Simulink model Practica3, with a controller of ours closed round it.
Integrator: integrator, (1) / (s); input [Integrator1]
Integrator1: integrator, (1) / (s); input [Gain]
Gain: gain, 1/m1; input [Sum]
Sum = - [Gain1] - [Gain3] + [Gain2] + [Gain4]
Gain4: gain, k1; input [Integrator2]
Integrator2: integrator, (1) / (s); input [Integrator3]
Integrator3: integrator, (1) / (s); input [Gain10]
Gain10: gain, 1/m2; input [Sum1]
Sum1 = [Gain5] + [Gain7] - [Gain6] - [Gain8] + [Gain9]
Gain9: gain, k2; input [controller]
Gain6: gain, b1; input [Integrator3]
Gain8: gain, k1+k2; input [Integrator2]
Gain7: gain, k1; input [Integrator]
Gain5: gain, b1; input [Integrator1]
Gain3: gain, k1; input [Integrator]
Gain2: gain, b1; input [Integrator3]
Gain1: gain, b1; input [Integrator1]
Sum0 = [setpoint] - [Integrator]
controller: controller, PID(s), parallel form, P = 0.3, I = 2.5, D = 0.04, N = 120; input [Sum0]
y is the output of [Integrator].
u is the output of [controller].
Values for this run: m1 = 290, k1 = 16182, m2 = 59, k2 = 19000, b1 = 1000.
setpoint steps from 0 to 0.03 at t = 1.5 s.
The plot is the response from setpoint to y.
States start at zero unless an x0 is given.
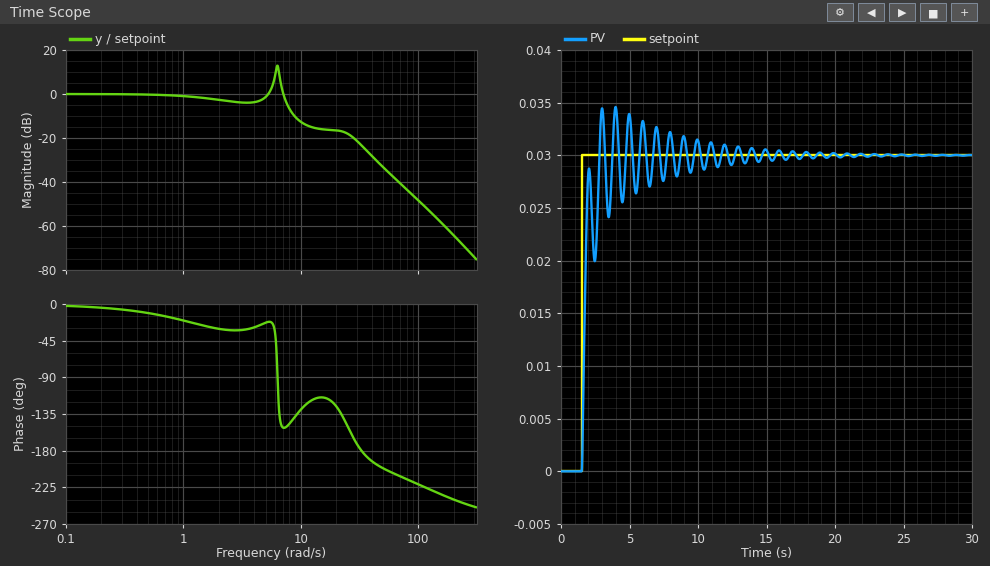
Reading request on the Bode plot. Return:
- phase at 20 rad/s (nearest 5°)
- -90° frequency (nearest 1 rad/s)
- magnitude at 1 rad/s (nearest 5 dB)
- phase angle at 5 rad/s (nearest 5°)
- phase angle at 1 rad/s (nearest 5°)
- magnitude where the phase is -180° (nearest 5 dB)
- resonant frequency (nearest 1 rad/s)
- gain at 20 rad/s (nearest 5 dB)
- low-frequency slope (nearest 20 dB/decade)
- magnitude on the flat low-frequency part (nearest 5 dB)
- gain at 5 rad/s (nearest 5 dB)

-125°
6 rad/s
0 dB
-25°
-20°
-25 dB
6 rad/s
-15 dB
0 dB/decade
0 dB
0 dB
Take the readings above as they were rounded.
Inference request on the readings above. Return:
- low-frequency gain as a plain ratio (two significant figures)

1.0
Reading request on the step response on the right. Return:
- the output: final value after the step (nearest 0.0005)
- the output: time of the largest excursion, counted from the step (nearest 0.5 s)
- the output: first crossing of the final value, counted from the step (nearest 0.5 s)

0.0300
2.5 s
1.5 s
